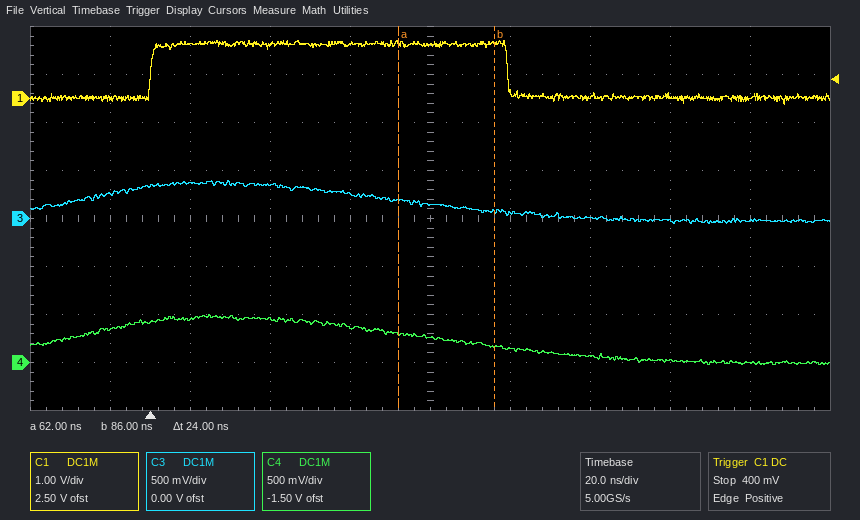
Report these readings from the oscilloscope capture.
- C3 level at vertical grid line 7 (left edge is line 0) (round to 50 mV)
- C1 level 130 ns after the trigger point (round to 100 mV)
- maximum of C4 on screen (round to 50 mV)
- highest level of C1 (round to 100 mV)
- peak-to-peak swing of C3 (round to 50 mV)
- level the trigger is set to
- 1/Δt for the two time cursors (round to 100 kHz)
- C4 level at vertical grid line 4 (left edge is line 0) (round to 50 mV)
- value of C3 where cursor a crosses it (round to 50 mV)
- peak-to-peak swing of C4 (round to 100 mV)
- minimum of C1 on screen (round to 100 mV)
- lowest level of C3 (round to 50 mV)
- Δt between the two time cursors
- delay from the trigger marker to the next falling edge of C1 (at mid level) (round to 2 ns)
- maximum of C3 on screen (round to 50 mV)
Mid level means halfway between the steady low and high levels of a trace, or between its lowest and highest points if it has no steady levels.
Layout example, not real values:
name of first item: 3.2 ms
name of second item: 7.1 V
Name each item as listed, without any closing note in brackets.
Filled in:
C3 level at vertical grid line 7 (left edge is line 0): 0 mV
C1 level 130 ns after the trigger point: 100 mV
maximum of C4 on screen: 500 mV
highest level of C1: 1.2 V
peak-to-peak swing of C3: 450 mV
level the trigger is set to: 400 mV
1/Δt for the two time cursors: 41.7 MHz
C4 level at vertical grid line 4 (left edge is line 0): 350 mV
value of C3 where cursor a crosses it: 200 mV
peak-to-peak swing of C4: 500 mV
minimum of C1 on screen: -100 mV
lowest level of C3: -50 mV
Δt between the two time cursors: 24 ns
delay from the trigger marker to the next falling edge of C1 (at mid level): 90 ns
maximum of C3 on screen: 400 mV
